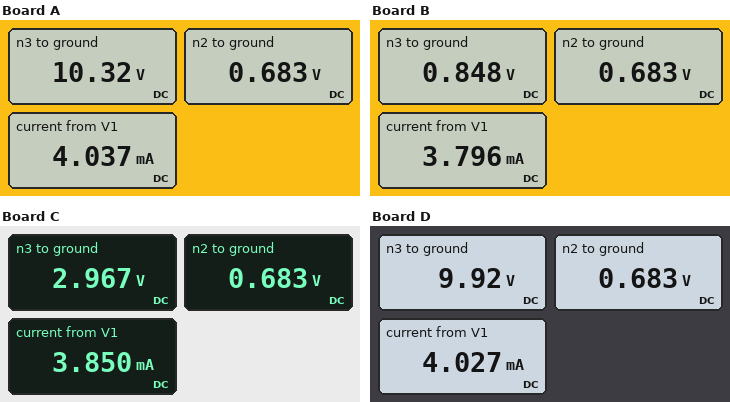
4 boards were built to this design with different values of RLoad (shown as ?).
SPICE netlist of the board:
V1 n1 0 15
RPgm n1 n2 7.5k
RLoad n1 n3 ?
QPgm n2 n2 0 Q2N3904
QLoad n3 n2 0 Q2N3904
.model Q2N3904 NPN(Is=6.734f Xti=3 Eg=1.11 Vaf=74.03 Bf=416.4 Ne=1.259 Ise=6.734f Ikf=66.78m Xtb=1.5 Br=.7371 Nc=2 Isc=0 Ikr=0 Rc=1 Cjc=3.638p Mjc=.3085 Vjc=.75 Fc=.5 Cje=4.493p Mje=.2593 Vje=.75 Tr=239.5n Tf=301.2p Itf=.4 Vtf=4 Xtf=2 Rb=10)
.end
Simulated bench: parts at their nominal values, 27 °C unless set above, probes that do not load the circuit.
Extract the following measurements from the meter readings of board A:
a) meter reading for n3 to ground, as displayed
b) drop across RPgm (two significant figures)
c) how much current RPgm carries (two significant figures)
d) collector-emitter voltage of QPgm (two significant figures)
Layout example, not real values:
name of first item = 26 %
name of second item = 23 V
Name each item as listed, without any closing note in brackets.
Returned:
meter reading for n3 to ground, as displayed = 10.32 V
drop across RPgm = 14 V
how much current RPgm carries = 1.9 mA
collector-emitter voltage of QPgm = 680 mV
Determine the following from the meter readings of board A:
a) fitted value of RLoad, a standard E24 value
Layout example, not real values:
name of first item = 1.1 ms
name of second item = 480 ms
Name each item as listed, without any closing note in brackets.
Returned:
fitted value of RLoad, a standard E24 value = 2.2 kΩ
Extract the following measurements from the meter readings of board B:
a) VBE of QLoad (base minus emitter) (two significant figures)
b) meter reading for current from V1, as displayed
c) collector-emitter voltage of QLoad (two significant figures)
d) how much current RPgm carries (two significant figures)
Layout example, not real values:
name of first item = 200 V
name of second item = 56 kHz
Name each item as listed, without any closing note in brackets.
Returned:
VBE of QLoad (base minus emitter) = 680 mV
meter reading for current from V1, as displayed = 3.796 mA
collector-emitter voltage of QLoad = 850 mV
how much current RPgm carries = 1.9 mA
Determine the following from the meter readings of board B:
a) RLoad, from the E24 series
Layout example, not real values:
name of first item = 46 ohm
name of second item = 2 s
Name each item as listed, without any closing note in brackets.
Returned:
RLoad, from the E24 series = 7.5 kΩ
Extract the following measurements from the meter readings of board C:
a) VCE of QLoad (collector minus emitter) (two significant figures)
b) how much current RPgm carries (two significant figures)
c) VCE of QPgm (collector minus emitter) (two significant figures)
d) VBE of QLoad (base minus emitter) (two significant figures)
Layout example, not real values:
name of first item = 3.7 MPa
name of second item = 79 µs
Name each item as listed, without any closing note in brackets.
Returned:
VCE of QLoad (collector minus emitter) = 3.0 V
how much current RPgm carries = 1.9 mA
VCE of QPgm (collector minus emitter) = 680 mV
VBE of QLoad (base minus emitter) = 680 mV
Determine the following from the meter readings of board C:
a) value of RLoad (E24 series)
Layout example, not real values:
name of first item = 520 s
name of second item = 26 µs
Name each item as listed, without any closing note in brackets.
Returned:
value of RLoad = 6.2 kΩ
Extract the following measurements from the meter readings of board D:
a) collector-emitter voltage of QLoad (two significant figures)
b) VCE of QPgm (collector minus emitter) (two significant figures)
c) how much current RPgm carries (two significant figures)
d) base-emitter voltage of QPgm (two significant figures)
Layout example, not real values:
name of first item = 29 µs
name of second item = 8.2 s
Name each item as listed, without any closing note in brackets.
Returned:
collector-emitter voltage of QLoad = 9.9 V
VCE of QPgm (collector minus emitter) = 680 mV
how much current RPgm carries = 1.9 mA
base-emitter voltage of QPgm = 680 mV
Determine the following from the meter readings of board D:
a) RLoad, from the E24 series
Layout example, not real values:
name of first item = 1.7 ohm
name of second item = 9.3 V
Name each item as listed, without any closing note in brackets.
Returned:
RLoad, from the E24 series = 2.4 kΩ
